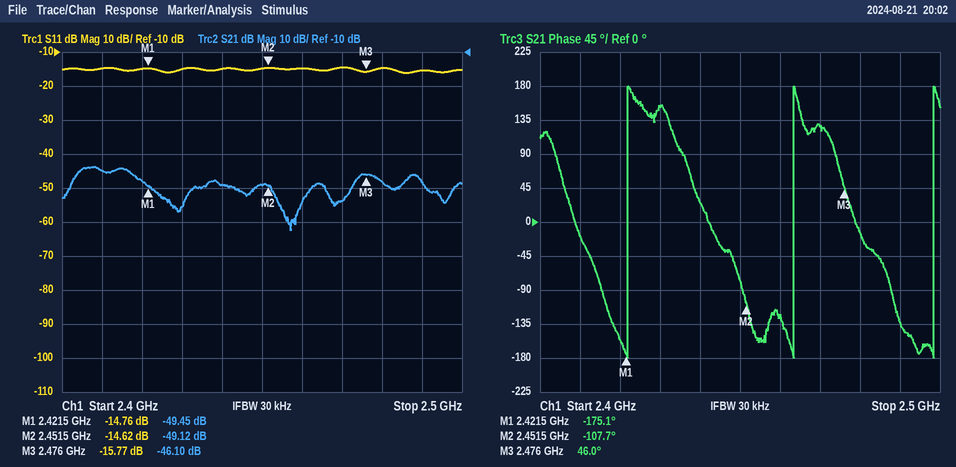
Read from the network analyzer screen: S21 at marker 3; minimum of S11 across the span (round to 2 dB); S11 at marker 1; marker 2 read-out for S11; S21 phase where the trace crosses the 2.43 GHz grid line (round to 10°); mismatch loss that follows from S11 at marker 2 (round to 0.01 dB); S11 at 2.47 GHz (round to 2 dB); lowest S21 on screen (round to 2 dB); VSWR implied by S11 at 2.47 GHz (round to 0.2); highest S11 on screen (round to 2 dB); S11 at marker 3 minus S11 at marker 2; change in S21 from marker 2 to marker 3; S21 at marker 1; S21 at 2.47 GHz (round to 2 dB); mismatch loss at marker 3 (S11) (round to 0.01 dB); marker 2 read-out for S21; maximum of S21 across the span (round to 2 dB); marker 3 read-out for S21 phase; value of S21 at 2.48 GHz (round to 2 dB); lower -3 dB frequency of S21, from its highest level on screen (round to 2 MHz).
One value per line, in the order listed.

-46.10 dB
-16 dB
-14.76 dB
-14.62 dB
150°
0.15 dB
-14 dB
-62 dB
1.4
-14 dB
-1.15 dB
3.02 dB
-49.45 dB
-54 dB
0.12 dB
-49.12 dB
-44 dB
46.0°
-48 dB
2.404 GHz
